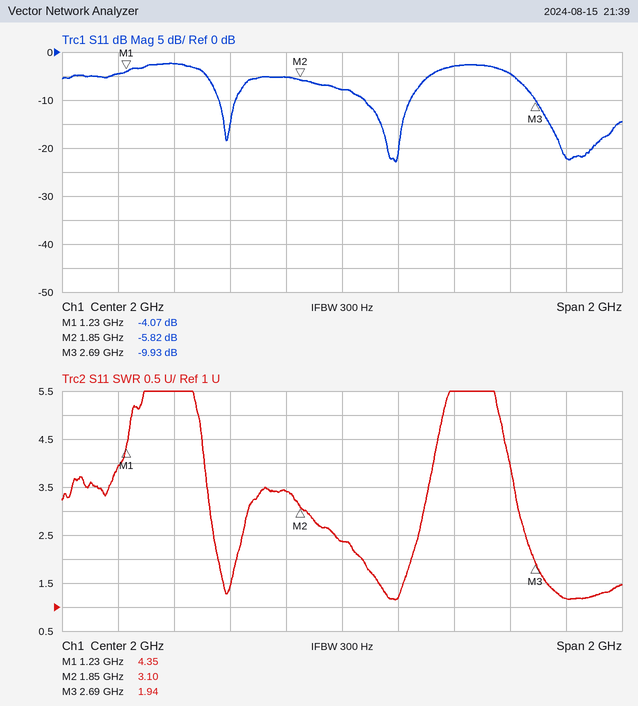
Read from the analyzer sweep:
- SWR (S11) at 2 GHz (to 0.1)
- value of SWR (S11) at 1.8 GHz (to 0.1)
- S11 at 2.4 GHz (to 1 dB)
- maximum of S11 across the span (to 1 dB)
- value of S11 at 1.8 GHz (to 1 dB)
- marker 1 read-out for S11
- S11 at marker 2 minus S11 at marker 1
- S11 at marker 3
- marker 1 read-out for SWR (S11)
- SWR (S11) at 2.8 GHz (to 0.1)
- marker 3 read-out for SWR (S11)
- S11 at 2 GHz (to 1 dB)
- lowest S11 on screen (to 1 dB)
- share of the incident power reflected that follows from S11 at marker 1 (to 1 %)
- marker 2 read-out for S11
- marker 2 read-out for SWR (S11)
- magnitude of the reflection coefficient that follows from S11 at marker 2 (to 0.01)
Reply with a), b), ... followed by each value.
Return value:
a) 2.4
b) 3.4
c) -3 dB
d) -2 dB
e) -5 dB
f) -4.07 dB
g) -1.75 dB
h) -9.93 dB
i) 4.35
j) 1.2
k) 1.94
l) -8 dB
m) -23 dB
n) 39 %
o) -5.82 dB
p) 3.10
q) 0.51
